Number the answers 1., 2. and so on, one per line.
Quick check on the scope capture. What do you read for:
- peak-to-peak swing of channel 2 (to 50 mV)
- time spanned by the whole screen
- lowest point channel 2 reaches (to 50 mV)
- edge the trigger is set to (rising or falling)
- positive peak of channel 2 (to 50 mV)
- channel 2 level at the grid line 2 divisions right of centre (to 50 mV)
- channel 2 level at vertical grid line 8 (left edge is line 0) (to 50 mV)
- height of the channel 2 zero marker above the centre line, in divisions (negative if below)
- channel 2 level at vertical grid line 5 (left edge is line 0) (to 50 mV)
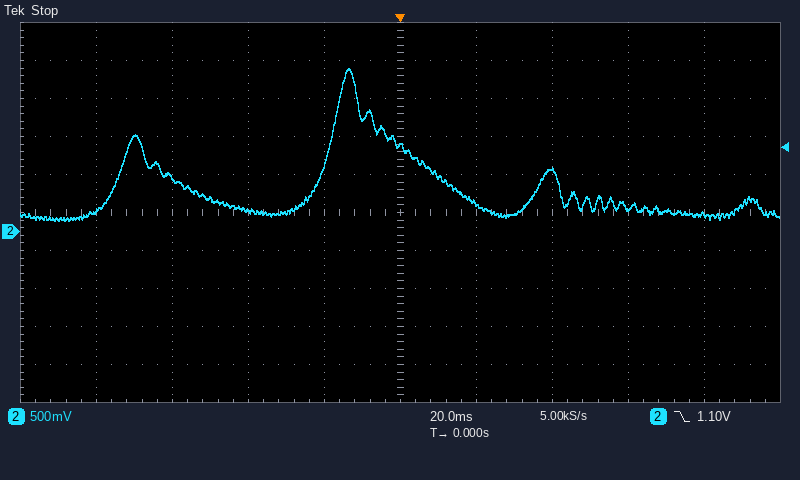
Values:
1. 2.00 V
2. 200 ms
3. 150 mV
4. falling
5. 2.15 V
6. 800 mV
7. 300 mV
8. -0.5 div
9. 1.10 V
